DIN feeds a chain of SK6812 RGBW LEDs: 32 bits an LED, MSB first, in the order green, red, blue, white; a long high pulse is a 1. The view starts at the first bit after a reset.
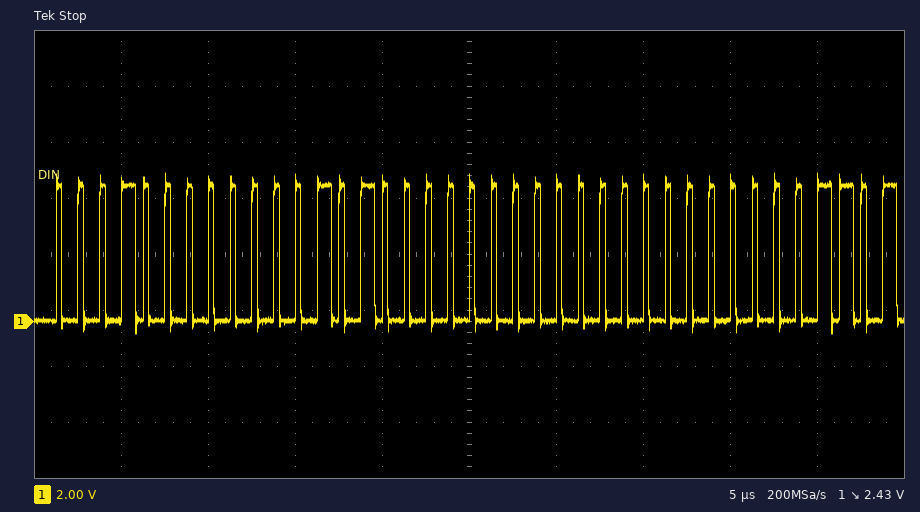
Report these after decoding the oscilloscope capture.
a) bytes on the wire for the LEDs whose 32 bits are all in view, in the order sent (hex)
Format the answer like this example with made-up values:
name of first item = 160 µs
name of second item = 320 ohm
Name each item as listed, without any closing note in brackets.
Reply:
bytes on the wire for the LEDs whose 32 bits are all in view, in the order sent = 10 0A 00 00
